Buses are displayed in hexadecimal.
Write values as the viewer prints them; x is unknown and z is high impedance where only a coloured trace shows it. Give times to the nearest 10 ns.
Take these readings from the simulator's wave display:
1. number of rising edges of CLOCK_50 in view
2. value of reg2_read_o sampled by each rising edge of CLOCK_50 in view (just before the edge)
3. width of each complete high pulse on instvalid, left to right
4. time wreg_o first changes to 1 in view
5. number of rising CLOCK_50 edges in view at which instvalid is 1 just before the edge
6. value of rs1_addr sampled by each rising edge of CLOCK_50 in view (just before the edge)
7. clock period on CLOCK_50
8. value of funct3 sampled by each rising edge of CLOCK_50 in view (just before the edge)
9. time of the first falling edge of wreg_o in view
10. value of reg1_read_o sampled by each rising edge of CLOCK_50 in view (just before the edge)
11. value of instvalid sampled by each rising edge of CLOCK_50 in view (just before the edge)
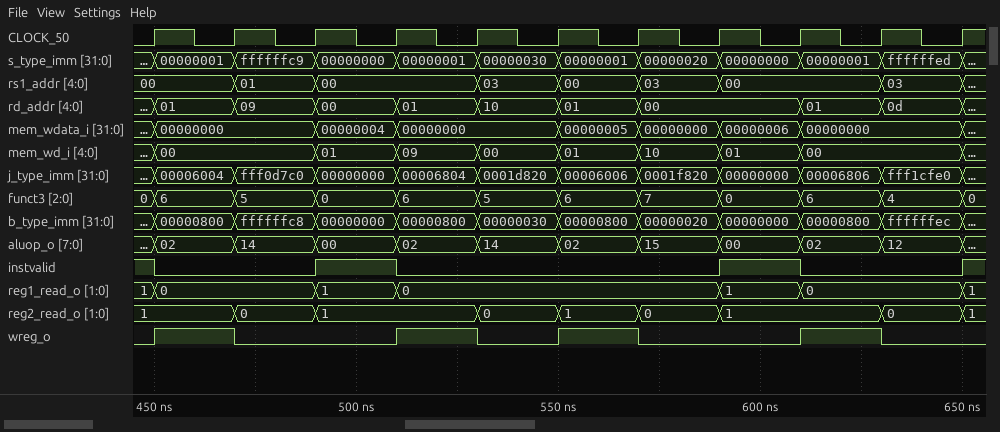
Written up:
11
1, 1, 0, 1, 1, 0, 1, 0, 1, 1, 0
20 ns, 20 ns
450 ns
3
00, 00, 01, 00, 00, 03, 00, 03, 00, 00, 03
20 ns
0, 6, 5, 0, 6, 5, 6, 7, 0, 6, 4
470 ns
1, 0, 0, 1, 0, 0, 0, 0, 1, 0, 0
1 0 0 1 0 0 0 0 1 0 0
